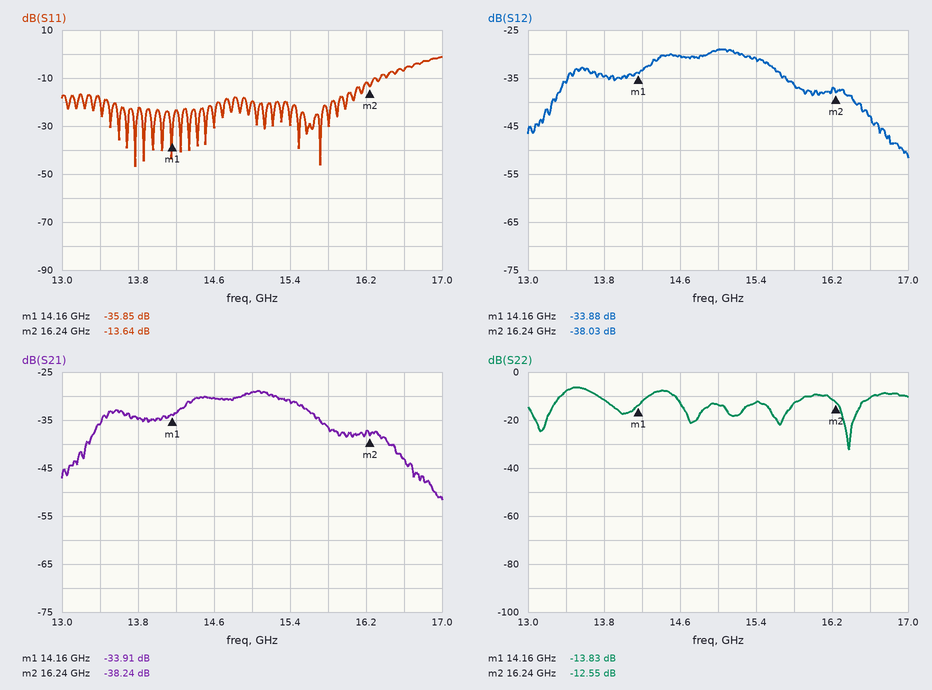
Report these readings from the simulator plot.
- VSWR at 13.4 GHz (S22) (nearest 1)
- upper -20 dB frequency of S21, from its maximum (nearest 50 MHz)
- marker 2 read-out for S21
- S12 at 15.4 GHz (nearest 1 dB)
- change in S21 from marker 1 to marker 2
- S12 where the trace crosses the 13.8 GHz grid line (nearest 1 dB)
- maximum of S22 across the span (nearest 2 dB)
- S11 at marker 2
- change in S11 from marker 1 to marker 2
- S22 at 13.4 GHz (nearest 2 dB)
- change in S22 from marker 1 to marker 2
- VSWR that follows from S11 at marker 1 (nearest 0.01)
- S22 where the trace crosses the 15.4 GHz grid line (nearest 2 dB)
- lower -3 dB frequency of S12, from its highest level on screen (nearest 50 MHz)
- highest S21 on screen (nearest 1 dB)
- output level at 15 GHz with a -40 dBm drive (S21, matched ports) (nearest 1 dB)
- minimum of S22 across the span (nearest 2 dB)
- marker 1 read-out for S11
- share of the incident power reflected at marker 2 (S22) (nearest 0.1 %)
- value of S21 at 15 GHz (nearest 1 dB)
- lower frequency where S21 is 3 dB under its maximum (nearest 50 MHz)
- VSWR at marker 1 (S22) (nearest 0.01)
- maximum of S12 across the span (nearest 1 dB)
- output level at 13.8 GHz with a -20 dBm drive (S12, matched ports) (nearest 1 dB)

2
16.90 GHz
-38.24 dB
-31 dB
-4.33 dB
-35 dB
-6 dB
-13.64 dB
22.21 dB
-8 dB
1.28 dB
1.03
-12 dB
14.30 GHz
-29 dB
-69 dBm
-32 dB
-35.85 dB
5.6 %
-29 dB
14.30 GHz
1.51
-29 dB
-55 dBm
